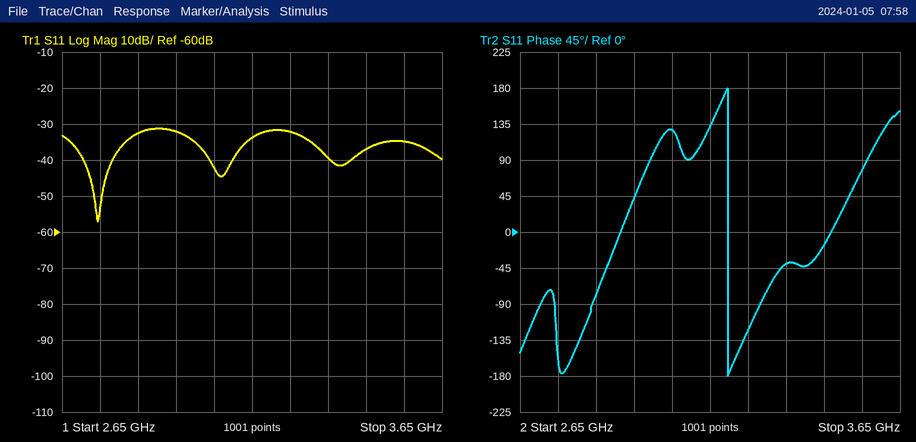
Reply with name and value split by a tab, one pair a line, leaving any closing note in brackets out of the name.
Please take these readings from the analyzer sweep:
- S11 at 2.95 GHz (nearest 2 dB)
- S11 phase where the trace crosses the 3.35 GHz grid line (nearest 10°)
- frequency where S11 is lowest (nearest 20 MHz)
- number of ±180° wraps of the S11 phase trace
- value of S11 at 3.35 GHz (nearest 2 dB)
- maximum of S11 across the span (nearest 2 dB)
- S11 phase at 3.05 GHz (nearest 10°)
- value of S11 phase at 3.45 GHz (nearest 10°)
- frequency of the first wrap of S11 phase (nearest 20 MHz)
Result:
S11 at 2.95 GHz	-32 dB
S11 phase where the trace crosses the 3.35 GHz grid line	-40°
frequency where S11 is lowest	2.74 GHz
number of ±180° wraps of the S11 phase trace	1
value of S11 at 3.35 GHz	-40 dB
maximum of S11 across the span	-32 dB
S11 phase at 3.05 GHz	130°
value of S11 phase at 3.45 GHz	-20°
frequency of the first wrap of S11 phase	3.20 GHz
